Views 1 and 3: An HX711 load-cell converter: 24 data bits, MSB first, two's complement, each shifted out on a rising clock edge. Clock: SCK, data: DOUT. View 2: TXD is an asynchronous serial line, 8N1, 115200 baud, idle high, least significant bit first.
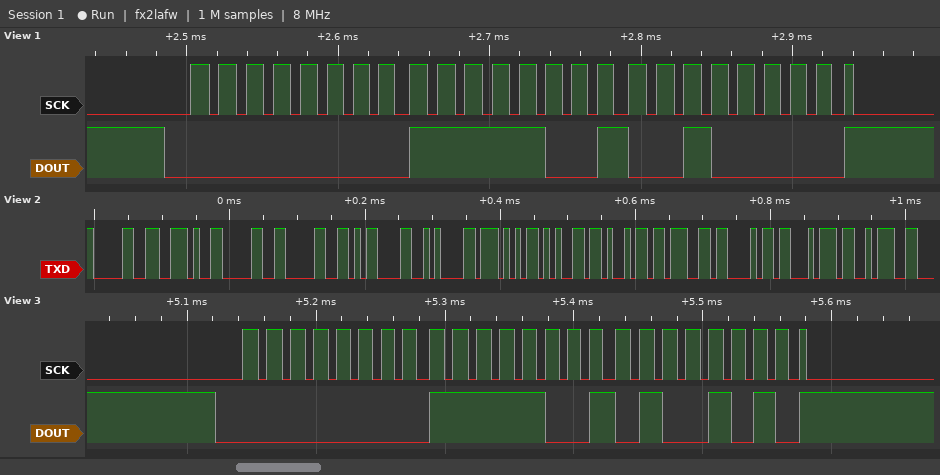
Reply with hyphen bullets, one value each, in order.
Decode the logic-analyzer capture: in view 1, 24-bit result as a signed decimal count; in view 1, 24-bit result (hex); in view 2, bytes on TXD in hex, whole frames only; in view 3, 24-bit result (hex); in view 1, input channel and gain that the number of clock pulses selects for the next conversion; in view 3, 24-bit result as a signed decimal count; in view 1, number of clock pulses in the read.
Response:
- 63776
- 0x00F920
- 30 2E 30 30 0D 0A 57 65 69 67 68 74 3A
- 0x00F94A
- channel A, gain 128
- 63818
- 25
